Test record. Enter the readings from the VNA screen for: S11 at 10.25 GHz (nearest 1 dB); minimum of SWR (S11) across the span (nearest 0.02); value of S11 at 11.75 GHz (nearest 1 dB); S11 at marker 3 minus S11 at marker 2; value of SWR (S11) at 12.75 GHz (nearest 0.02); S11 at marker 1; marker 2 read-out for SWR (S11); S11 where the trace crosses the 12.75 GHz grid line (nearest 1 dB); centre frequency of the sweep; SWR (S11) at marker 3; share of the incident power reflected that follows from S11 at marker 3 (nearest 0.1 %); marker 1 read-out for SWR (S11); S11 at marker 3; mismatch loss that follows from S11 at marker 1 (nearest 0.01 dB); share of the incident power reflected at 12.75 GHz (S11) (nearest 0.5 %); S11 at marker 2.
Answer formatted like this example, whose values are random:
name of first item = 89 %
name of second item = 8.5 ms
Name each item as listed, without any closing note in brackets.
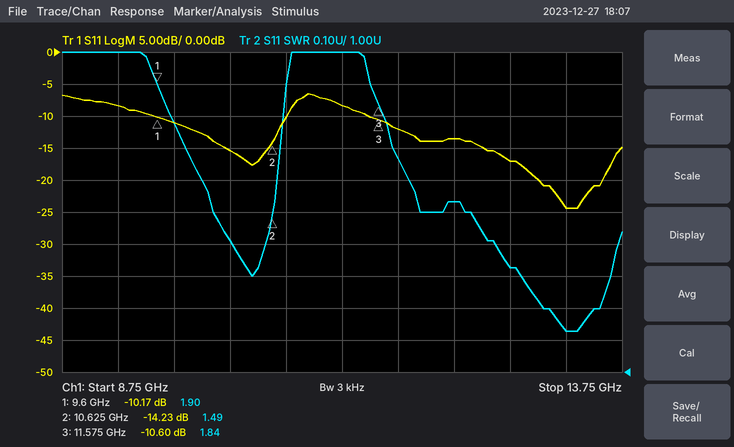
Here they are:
S11 at 10.25 GHz = -15 dB
minimum of SWR (S11) across the span = 1.12
value of S11 at 11.75 GHz = -12 dB
S11 at marker 3 minus S11 at marker 2 = 3.63 dB
value of SWR (S11) at 12.75 GHz = 1.32
S11 at marker 1 = -10.17 dB
marker 2 read-out for SWR = 1.49
S11 where the trace crosses the 12.75 GHz grid line = -17 dB
centre frequency of the sweep = 11.25 GHz
SWR (S11) at marker 3 = 1.84
share of the incident power reflected that follows from S11 at marker 3 = 8.7 %
marker 1 read-out for SWR = 1.90
S11 at marker 3 = -10.60 dB
mismatch loss that follows from S11 at marker 1 = 0.44 dB
share of the incident power reflected at 12.75 GHz (S11) = 2.0 %
S11 at marker 2 = -14.23 dB
